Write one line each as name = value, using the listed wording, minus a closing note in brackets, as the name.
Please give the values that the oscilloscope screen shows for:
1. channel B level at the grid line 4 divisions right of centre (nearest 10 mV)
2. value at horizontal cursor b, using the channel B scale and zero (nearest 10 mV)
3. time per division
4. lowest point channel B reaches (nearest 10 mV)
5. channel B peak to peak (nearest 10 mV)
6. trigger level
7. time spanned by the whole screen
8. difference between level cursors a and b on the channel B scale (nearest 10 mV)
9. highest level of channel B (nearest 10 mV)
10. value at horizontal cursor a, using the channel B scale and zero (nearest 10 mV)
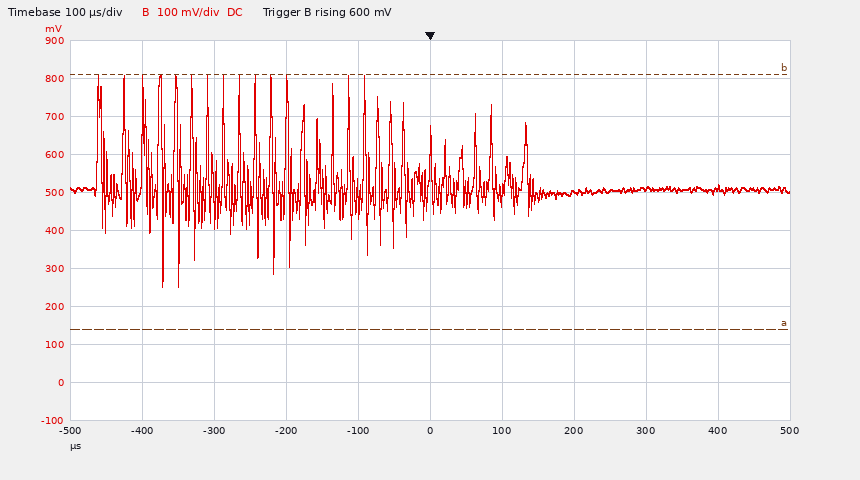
channel B level at the grid line 4 divisions right of centre = 510 mV
value at horizontal cursor b, using the channel B scale and zero = 810 mV
time per division = 100 µs
lowest point channel B reaches = 250 mV
channel B peak to peak = 560 mV
trigger level = 600 mV
time spanned by the whole screen = 1 ms
difference between level cursors a and b on the channel B scale = 670 mV
highest level of channel B = 810 mV
value at horizontal cursor a, using the channel B scale and zero = 140 mV
